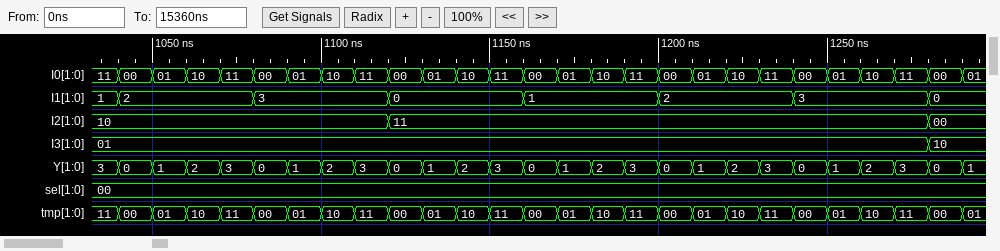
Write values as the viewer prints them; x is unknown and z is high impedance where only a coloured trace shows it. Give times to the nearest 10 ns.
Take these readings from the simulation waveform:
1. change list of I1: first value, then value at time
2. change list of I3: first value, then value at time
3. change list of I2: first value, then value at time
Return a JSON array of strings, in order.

["1, 2 at 1040 ns, 3 at 1080 ns, 0 at 1120 ns, 1 at 1160 ns, 2 at 1200 ns, 3 at 1240 ns, 0 at 1280 ns", "01, 10 at 1280 ns", "10, 11 at 1120 ns, 00 at 1280 ns"]
